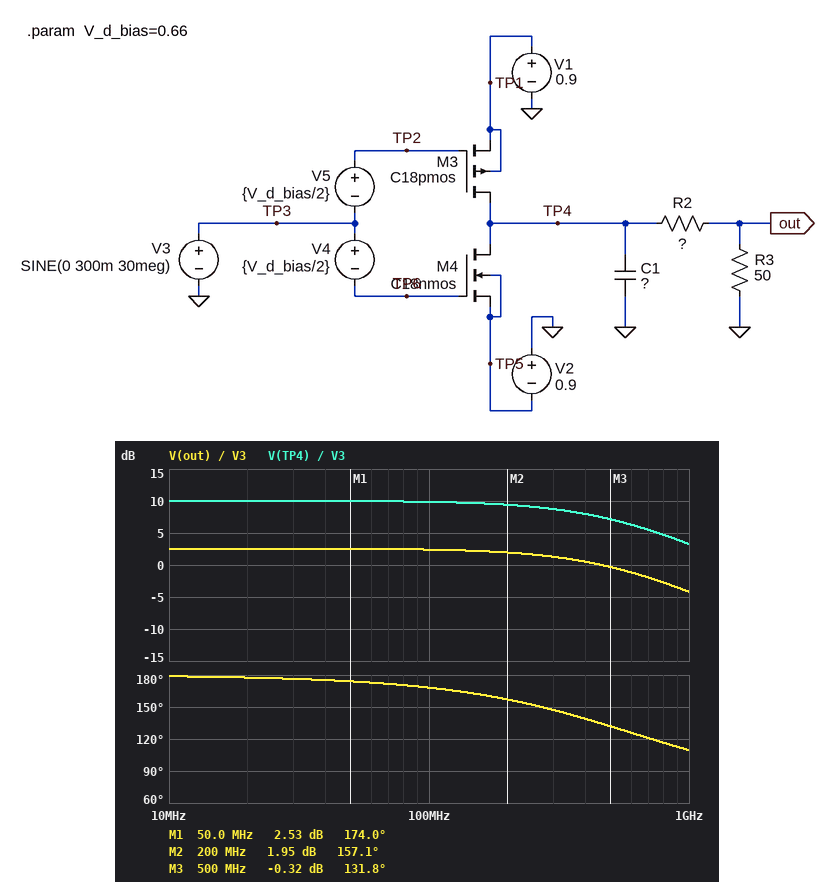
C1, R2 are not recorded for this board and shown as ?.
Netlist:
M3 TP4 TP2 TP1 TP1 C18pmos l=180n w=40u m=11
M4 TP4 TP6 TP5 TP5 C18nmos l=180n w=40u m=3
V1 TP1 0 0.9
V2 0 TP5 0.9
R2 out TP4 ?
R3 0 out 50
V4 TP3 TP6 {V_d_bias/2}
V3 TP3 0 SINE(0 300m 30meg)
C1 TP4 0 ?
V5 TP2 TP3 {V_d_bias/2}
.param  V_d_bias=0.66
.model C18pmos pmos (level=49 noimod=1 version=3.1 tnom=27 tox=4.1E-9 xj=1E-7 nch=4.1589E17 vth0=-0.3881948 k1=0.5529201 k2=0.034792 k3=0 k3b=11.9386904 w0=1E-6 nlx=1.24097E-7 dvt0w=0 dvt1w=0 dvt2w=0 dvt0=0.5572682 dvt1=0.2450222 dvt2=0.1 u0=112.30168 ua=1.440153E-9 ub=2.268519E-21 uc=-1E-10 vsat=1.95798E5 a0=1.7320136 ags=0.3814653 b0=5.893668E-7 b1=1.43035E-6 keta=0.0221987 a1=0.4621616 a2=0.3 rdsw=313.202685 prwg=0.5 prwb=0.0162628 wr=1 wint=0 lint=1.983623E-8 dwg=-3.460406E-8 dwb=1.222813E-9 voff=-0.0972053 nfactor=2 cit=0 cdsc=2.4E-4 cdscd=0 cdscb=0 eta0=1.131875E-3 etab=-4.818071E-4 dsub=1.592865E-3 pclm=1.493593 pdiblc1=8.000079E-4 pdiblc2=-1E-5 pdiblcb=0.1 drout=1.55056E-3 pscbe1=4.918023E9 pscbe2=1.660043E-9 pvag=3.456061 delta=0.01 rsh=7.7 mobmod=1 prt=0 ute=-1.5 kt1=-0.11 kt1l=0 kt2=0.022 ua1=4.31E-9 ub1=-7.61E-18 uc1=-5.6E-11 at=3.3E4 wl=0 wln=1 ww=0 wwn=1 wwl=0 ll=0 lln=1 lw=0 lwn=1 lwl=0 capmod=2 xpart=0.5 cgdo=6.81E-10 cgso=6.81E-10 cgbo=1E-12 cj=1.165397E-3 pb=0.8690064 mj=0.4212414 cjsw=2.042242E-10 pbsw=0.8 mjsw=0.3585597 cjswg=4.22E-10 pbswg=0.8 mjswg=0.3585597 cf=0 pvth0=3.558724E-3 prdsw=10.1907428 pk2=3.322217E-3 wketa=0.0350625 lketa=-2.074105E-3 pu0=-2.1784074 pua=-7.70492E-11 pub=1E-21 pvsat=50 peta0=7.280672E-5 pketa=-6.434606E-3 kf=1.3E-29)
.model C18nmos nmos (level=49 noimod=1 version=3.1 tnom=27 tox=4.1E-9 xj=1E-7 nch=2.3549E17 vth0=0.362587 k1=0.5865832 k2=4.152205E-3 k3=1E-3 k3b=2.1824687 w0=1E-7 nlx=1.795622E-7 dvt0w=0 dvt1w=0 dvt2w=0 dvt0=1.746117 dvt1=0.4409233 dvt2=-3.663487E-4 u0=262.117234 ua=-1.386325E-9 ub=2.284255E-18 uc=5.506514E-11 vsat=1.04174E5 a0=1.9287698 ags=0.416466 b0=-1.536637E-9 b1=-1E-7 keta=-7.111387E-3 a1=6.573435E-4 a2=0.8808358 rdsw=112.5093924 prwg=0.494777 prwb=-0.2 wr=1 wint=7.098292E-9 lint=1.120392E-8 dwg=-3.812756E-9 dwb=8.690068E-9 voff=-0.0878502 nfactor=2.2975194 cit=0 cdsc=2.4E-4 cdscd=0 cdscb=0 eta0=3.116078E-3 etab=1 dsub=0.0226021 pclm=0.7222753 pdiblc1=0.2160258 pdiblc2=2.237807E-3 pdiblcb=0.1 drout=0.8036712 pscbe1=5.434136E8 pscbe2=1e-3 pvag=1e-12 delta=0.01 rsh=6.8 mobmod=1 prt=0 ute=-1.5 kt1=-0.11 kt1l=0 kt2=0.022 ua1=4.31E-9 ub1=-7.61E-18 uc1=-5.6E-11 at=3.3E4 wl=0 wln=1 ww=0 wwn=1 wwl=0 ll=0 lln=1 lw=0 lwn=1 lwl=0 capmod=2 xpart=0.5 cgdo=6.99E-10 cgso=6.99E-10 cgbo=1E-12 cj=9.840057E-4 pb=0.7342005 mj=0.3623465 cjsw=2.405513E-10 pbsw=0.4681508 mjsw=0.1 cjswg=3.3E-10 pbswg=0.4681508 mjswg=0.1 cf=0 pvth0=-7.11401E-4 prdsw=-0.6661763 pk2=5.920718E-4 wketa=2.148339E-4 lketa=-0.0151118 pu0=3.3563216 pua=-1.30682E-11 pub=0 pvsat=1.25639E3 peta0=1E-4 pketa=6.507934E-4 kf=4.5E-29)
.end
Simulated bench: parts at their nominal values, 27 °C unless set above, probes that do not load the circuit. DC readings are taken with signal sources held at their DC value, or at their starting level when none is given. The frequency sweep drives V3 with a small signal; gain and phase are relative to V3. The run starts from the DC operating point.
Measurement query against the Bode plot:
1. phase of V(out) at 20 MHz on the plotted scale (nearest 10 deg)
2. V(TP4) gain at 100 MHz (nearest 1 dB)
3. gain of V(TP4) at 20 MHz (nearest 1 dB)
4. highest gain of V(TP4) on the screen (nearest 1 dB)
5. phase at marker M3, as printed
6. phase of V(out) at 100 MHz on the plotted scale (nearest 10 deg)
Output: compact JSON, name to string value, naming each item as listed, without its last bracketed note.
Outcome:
{"phase of V(out) at 20 MHz on the plotted scale": "180 deg", "V(TP4) gain at 100 MHz": "10 dB", "gain of V(TP4) at 20 MHz": "10 dB", "highest gain of V(TP4) on the screen": "10 dB", "phase at marker M3, as printed": "131.8 deg", "phase of V(out) at 100 MHz on the plotted scale": "170 deg"}
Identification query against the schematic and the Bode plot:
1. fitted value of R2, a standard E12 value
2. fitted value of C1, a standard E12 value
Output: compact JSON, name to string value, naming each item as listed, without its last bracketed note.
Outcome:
{"fitted value of R2, a standard E12 value": "68 Ω", "fitted value of C1, a standard E12 value": "2.2 pF"}
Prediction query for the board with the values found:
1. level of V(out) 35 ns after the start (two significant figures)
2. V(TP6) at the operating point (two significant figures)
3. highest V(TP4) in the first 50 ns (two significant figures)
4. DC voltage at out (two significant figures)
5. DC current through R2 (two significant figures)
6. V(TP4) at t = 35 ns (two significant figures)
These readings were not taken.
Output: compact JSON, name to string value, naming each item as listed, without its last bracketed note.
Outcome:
{"level of V(out) 35 ns after the start": "-100 mV", "V(TP6) at the operating point": "-330 mV", "highest V(TP4) in the first 50 ns": "770 mV", "DC voltage at out": "-3.5 mV", "DC current through R2": "70 µA", "V(TP4) at t = 35 ns": "-250 mV"}
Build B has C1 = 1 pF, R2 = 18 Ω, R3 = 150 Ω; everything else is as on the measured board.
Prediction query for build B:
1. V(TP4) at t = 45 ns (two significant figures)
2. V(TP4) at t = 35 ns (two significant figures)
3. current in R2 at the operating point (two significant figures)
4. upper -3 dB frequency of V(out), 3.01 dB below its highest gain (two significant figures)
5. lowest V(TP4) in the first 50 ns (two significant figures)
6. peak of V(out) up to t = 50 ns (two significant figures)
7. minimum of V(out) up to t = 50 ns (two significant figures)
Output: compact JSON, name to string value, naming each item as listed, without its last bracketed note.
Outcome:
{"V(TP4) at t = 45 ns": "-780 mV", "V(TP4) at t = 35 ns": "-360 mV", "current in R2 at the operating point": "69 µA", "upper -3 dB frequency of V(out), 3.01 dB below its highest gain": "650 MHz", "lowest V(TP4) in the first 50 ns": "-800 mV", "peak of V(out) up to t = 50 ns": "720 mV", "minimum of V(out) up to t = 50 ns": "-710 mV"}
